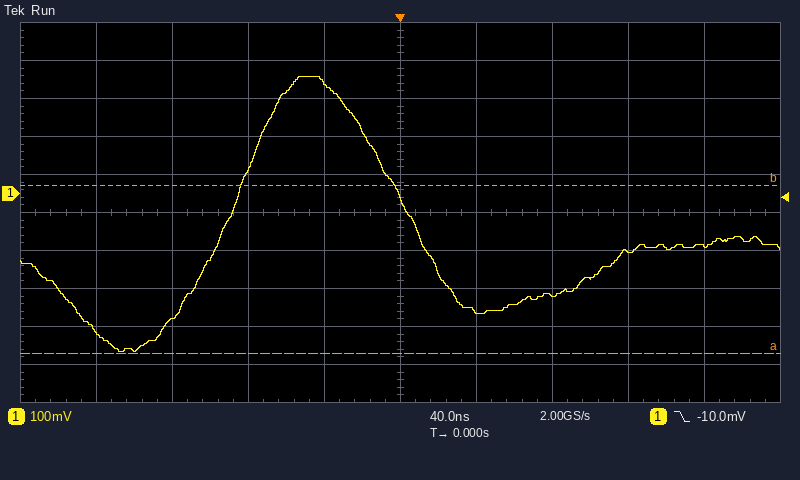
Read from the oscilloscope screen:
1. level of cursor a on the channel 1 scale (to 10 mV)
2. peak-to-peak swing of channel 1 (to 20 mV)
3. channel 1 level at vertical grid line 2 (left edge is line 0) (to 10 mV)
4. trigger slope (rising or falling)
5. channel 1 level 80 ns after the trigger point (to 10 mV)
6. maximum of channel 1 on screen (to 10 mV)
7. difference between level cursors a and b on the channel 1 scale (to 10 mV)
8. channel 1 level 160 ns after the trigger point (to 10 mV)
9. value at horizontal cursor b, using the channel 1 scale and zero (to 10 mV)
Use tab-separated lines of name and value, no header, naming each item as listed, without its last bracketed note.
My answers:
level of cursor a on the channel 1 scale	-420 mV
peak-to-peak swing of channel 1	720 mV
channel 1 level at vertical grid line 2 (left edge is line 0)	-330 mV
trigger slope	falling
channel 1 level 80 ns after the trigger point	-270 mV
maximum of channel 1 on screen	310 mV
difference between level cursors a and b on the channel 1 scale	440 mV
channel 1 level 160 ns after the trigger point	-140 mV
value at horizontal cursor b, using the channel 1 scale and zero	20 mV
